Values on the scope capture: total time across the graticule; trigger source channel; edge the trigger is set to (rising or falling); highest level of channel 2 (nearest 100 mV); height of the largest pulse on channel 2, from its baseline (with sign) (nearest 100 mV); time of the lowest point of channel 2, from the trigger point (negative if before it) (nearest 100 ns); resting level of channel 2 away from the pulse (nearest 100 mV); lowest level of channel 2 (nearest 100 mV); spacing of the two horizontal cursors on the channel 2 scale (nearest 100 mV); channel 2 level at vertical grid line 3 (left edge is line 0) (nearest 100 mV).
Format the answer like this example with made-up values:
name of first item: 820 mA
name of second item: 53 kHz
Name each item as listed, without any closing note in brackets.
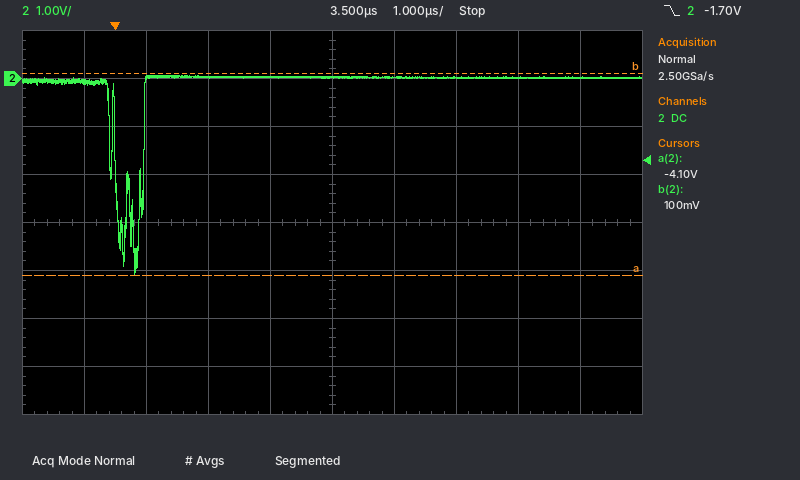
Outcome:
total time across the graticule: 10 µs
trigger source channel: channel 2
edge the trigger is set to: falling
highest level of channel 2: 100 mV
height of the largest pulse on channel 2, from its baseline (with sign): -4.1 V
time of the lowest point of channel 2, from the trigger point (negative if before it): +300 ns
resting level of channel 2 away from the pulse: 0.0 V
lowest level of channel 2: -4.1 V
spacing of the two horizontal cursors on the channel 2 scale: 4.2 V
channel 2 level at vertical grid line 3 (left edge is line 0): 0.0 V
